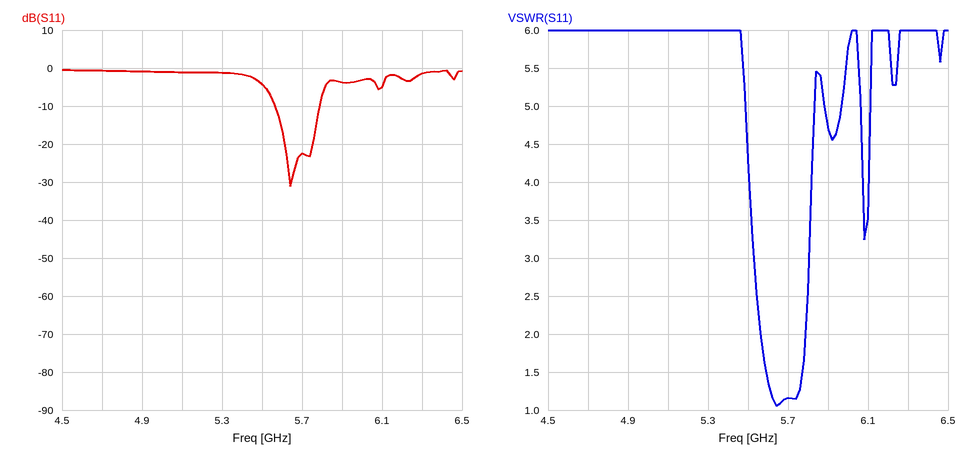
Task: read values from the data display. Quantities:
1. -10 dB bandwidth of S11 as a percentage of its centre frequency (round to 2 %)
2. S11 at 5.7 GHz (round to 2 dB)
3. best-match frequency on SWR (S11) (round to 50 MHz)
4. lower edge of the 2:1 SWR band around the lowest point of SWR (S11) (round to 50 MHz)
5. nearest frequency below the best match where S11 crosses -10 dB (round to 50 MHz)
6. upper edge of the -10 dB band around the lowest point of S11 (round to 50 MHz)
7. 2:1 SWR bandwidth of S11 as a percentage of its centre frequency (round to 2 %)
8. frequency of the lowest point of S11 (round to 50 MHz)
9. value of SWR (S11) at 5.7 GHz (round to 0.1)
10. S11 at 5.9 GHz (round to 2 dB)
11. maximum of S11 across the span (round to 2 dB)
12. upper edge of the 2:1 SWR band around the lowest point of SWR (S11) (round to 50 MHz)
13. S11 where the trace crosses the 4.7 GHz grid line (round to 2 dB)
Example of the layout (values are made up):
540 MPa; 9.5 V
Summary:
4 %; -22 dB; 5.65 GHz; 5.55 GHz; 5.55 GHz; 5.80 GHz; 4 %; 5.65 GHz; 1.2; -4 dB; 0 dB; 5.80 GHz; 0 dB
